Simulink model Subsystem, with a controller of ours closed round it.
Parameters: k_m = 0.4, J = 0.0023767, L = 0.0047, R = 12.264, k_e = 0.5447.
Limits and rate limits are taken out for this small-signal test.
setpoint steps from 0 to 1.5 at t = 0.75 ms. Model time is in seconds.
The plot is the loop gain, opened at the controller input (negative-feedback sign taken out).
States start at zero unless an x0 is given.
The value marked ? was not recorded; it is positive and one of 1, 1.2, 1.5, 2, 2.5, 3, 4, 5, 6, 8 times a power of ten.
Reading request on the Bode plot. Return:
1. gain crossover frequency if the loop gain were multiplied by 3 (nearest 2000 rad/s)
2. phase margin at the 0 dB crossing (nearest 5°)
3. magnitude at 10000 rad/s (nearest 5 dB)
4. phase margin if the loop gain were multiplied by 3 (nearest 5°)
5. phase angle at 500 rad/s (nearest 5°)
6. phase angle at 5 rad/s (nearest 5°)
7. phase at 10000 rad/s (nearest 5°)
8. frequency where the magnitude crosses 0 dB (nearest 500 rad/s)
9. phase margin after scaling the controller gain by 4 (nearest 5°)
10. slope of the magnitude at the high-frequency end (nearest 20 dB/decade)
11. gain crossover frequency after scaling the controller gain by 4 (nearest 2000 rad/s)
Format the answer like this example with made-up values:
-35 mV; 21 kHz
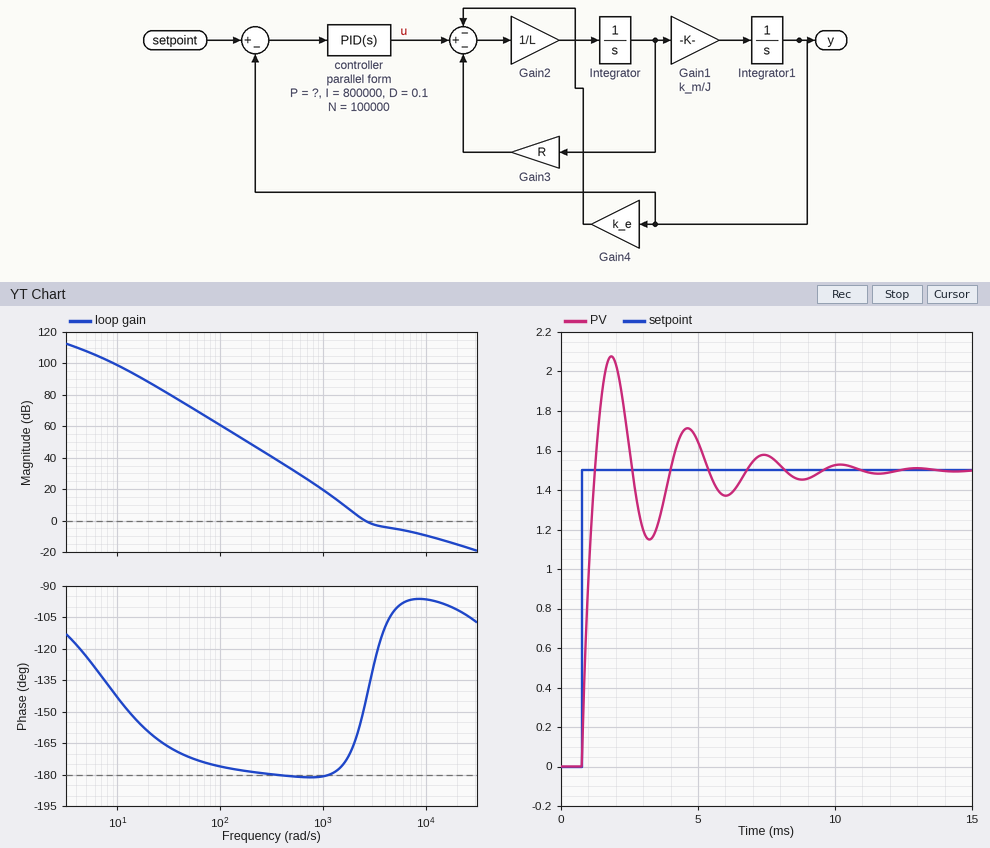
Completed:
10000 rad/s; 35°; -10 dB; 85°; -180°; -125°; -95°; 2500 rad/s; 80°; -20 dB/decade; 14000 rad/s
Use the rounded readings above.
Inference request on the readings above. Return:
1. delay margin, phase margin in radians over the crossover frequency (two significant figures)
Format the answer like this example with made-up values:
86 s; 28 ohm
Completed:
0.00024 s
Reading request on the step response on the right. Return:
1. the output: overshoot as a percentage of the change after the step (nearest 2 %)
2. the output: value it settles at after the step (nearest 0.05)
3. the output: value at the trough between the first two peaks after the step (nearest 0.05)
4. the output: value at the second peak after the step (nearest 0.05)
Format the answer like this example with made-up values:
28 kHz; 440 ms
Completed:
38 %; 1.50; 1.15; 1.70
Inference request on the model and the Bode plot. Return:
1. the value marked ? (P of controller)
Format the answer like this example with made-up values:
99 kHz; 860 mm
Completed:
250
